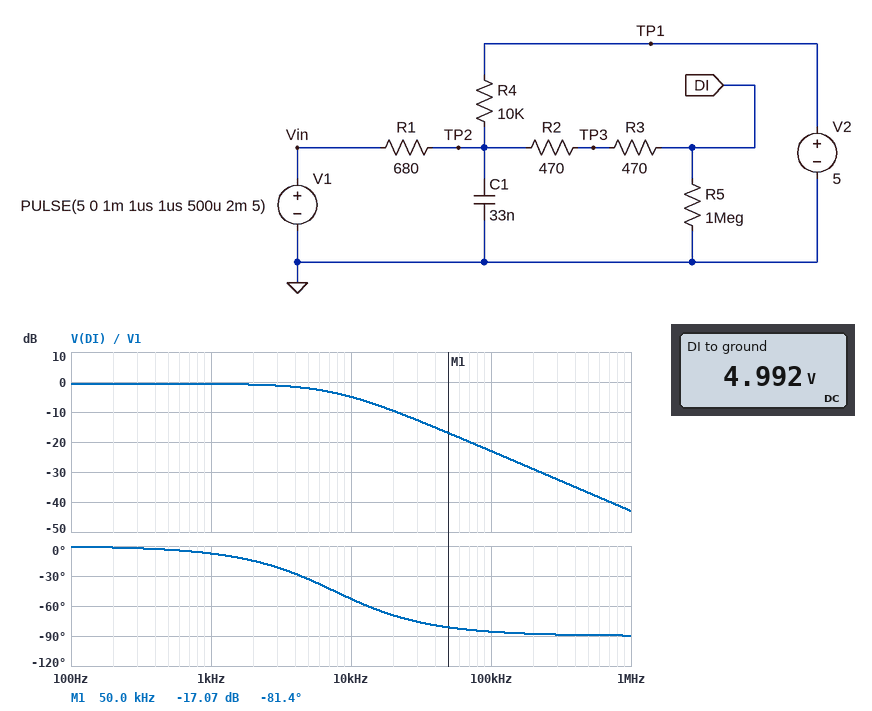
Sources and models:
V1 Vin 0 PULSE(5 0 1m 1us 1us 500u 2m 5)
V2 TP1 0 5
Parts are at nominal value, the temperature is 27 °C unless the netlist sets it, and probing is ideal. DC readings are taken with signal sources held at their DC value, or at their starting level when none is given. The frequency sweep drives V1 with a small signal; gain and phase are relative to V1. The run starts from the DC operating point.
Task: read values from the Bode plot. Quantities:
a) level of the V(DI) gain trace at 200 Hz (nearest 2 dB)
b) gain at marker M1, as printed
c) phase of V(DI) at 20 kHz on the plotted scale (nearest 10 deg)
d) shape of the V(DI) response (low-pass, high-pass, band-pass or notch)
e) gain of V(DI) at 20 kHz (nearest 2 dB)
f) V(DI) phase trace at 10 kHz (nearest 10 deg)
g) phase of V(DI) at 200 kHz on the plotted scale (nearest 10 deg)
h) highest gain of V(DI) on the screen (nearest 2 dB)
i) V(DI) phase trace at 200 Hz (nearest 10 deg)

0 dB
-17.07 dB
-70 deg
low-pass
-10 dB
-50 deg
-90 deg
0 dB
0 deg
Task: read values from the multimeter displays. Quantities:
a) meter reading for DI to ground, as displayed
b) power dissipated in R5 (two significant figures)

4.992 V
25 µW
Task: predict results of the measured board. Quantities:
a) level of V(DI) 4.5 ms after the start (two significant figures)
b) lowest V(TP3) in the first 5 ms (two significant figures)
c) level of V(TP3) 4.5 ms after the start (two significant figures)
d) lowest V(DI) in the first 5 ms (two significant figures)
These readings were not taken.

5.0 V
320 mV
5.0 V
320 mV
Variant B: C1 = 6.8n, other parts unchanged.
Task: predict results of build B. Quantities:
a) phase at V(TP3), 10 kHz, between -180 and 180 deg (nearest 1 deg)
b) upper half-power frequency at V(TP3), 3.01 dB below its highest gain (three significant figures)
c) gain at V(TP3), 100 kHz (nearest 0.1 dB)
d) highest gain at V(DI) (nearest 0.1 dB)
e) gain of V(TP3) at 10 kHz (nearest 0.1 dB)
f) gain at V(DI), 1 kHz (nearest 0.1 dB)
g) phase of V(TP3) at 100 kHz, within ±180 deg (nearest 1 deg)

-15 deg
36.8 kHz
-9.8 dB
-0.6 dB
-0.9 dB
-0.6 dB
-70 deg
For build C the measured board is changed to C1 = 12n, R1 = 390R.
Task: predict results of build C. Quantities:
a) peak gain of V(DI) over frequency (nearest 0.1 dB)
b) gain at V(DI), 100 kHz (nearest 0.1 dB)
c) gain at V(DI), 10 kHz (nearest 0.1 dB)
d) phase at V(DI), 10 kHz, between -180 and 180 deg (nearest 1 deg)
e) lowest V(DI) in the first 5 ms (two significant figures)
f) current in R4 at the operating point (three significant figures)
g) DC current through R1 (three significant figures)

-0.3 dB
-9.9 dB
-0.7 dB
-16 deg
190 mV
187 nA
4.81 µA
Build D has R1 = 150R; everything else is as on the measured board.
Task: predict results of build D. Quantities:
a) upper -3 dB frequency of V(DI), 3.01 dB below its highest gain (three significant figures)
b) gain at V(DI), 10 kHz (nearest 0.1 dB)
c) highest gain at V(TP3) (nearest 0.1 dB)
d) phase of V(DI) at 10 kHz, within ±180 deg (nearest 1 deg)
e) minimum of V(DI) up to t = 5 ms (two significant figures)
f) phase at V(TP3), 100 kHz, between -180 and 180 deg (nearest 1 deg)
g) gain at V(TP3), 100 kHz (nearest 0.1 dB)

32.6 kHz
-0.5 dB
-0.1 dB
-17 deg
74 mV
-72 deg
-10.3 dB
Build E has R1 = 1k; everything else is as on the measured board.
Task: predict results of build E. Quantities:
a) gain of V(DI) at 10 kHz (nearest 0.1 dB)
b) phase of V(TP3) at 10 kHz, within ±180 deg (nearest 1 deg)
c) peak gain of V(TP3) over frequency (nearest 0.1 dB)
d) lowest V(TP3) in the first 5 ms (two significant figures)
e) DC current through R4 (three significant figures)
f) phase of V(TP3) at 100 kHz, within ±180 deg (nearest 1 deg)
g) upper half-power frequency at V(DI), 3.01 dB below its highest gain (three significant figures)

-7.4 dB
-62 deg
-0.8 dB
450 mV
454 nA
-87 deg
5.31 kHz
